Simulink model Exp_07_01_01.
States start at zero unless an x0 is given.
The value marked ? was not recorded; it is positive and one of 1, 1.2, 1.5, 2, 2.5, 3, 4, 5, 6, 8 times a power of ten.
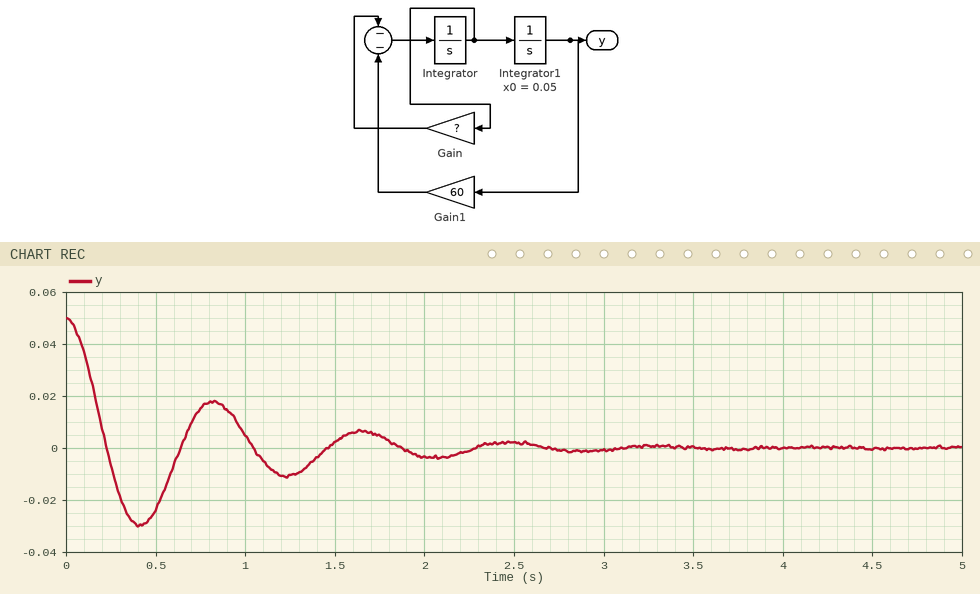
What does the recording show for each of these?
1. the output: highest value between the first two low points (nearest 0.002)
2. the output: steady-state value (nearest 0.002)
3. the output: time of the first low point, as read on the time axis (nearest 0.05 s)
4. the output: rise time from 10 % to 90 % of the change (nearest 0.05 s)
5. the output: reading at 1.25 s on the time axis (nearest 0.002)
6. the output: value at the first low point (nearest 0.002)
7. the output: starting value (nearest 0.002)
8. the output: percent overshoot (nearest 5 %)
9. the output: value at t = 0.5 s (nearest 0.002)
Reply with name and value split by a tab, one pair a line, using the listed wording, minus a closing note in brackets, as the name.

the output: highest value between the first two low points	0.018
the output: steady-state value	0.000
the output: time of the first low point, as read on the time axis	0.40 s
the output: rise time from 10 % to 90 % of the change	0.15 s
the output: reading at 1.25 s on the time axis	-0.010
the output: value at the first low point	-0.030
the output: starting value	0.050
the output: percent overshoot	60 %
the output: value at t = 0.5 s	-0.024
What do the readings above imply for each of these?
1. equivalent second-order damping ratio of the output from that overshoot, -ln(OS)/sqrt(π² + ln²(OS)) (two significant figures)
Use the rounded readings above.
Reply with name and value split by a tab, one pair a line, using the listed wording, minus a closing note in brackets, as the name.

equivalent second-order damping ratio of the output from that overshoot, -ln(OS)/sqrt(π² + ln²(OS))	0.16
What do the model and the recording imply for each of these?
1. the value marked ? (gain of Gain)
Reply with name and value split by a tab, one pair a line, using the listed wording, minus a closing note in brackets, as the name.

the value marked ?	2.5
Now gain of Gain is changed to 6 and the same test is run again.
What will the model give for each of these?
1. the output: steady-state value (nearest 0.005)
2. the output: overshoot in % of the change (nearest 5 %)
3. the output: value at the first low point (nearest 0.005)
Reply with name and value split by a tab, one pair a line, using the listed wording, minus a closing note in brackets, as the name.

the output: steady-state value	0.000
the output: overshoot in % of the change	25 %
the output: value at the first low point	-0.015
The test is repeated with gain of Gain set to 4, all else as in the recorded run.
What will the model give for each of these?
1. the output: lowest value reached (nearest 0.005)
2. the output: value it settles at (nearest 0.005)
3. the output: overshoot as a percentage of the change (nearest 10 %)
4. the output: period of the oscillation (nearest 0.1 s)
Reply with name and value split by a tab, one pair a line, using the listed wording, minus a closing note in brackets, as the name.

the output: lowest value reached	-0.020
the output: value it settles at	0.000
the output: overshoot as a percentage of the change	40 %
the output: period of the oscillation	0.8 s
